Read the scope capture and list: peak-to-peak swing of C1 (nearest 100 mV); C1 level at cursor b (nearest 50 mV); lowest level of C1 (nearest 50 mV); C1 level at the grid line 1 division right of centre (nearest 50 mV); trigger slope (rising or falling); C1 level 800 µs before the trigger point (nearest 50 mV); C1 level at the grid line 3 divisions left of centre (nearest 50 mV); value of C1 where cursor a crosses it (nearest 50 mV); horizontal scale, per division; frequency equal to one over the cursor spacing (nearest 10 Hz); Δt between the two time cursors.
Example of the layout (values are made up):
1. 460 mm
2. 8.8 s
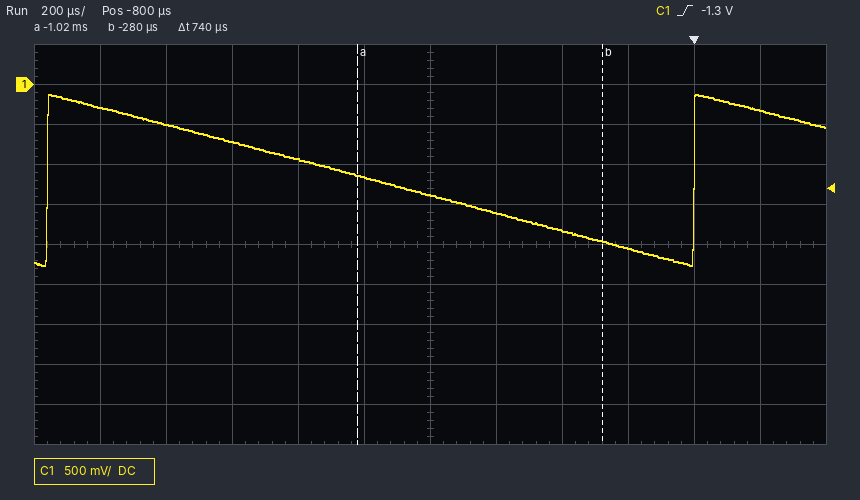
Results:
1. 2.10 V
2. -1.95 V
3. -2.25 V
4. -1.60 V
5. rising
6. -1.40 V
7. -700 mV
8. -1.15 V
9. 200 µs
10. 1.35 kHz
11. 740 µs
